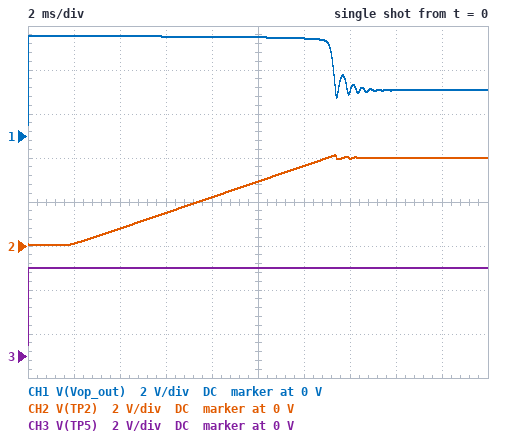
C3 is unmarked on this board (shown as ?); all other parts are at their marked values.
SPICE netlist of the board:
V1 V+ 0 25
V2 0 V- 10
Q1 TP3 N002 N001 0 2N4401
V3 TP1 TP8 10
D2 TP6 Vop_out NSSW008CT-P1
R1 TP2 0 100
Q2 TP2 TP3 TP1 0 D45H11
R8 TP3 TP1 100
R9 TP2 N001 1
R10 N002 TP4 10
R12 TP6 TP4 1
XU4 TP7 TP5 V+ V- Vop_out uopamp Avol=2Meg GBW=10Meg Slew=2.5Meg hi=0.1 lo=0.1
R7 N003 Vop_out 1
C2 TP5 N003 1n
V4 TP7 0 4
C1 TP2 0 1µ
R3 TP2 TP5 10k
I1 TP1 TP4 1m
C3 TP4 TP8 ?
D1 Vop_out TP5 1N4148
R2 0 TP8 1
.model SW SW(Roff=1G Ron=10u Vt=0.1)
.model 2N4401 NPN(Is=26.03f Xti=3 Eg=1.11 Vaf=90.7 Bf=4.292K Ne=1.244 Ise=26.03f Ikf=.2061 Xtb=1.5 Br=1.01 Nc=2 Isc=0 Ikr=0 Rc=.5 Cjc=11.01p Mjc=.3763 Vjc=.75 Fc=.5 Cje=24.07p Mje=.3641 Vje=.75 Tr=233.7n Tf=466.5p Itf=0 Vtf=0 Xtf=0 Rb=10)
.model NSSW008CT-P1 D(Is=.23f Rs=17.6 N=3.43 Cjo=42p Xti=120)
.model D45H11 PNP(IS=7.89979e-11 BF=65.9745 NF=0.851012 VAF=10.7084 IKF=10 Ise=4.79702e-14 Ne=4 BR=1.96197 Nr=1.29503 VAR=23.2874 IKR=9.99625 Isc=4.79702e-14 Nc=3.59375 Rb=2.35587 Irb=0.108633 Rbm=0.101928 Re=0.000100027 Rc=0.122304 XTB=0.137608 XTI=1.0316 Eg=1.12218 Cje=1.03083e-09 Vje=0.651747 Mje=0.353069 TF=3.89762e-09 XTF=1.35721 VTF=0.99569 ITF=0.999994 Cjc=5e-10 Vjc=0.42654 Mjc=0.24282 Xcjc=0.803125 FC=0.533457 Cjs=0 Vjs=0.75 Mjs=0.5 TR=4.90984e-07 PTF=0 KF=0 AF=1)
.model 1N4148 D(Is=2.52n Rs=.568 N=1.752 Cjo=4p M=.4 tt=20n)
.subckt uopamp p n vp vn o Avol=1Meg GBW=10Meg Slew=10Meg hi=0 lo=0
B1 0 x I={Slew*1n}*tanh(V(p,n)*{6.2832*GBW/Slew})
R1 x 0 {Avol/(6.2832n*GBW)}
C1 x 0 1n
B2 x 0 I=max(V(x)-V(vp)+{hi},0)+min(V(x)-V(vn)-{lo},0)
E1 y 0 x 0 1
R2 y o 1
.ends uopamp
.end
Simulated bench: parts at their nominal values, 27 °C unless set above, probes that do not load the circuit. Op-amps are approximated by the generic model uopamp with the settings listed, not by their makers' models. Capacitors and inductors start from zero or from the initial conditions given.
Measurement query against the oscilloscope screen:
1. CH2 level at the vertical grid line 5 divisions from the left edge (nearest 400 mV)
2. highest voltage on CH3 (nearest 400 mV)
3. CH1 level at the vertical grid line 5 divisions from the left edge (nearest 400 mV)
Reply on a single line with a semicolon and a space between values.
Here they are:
2.8 V; 4.0 V; 4.4 V
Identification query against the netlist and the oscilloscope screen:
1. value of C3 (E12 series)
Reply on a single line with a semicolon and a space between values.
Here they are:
2.7 µF
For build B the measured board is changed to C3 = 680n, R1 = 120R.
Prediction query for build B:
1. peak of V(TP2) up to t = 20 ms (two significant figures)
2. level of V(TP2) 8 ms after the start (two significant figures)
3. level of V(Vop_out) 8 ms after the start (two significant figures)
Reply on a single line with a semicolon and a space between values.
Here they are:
4.2 V; 4.0 V; 2.1 V
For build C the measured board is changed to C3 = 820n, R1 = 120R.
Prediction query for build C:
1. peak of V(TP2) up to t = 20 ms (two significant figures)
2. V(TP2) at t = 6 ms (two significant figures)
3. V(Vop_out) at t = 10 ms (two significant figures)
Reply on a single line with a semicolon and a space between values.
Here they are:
4.2 V; 4.0 V; 2.1 V
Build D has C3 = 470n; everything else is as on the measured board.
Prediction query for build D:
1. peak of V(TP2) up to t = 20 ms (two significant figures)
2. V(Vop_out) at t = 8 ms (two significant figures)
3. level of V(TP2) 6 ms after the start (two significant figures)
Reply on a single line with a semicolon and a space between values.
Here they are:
4.3 V; 2.1 V; 4.0 V
